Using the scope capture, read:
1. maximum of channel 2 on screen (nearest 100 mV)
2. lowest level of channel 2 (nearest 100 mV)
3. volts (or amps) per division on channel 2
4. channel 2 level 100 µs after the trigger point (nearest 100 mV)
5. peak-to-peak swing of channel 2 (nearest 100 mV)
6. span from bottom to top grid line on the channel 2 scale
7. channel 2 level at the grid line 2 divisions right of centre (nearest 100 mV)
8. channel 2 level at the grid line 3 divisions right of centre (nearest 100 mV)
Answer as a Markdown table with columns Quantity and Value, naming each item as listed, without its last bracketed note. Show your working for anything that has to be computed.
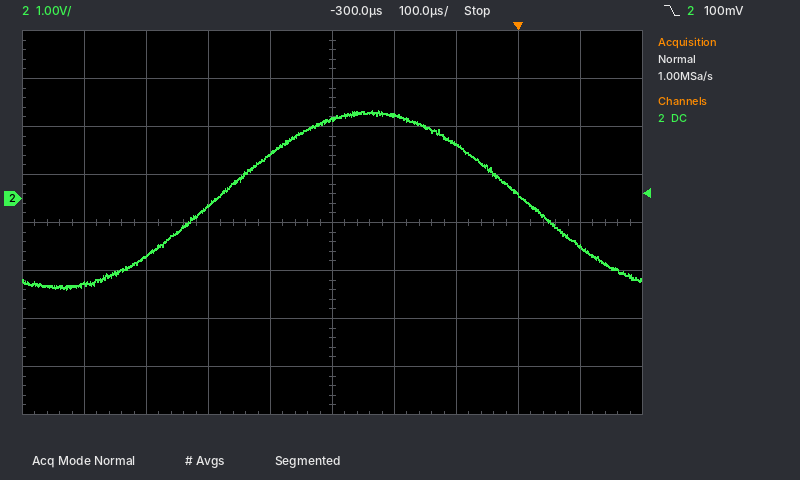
| Quantity | Value |
|---|---|
| maximum of channel 2 on screen | 1.8 V |
| lowest level of channel 2 | -1.9 V |
| volts (or amps) per division on channel 2 | 1 V |
| channel 2 level 100 µs after the trigger point | -1.0 V |
| peak-to-peak swing of channel 2 | 1.8 V − (-1.9 V) = 3.7 V |
| span from bottom to top grid line on the channel 2 scale | 8 V |
| channel 2 level at the grid line 2 divisions right of centre | 1.1 V |
| channel 2 level at the grid line 3 divisions right of centre | 100 mV |
